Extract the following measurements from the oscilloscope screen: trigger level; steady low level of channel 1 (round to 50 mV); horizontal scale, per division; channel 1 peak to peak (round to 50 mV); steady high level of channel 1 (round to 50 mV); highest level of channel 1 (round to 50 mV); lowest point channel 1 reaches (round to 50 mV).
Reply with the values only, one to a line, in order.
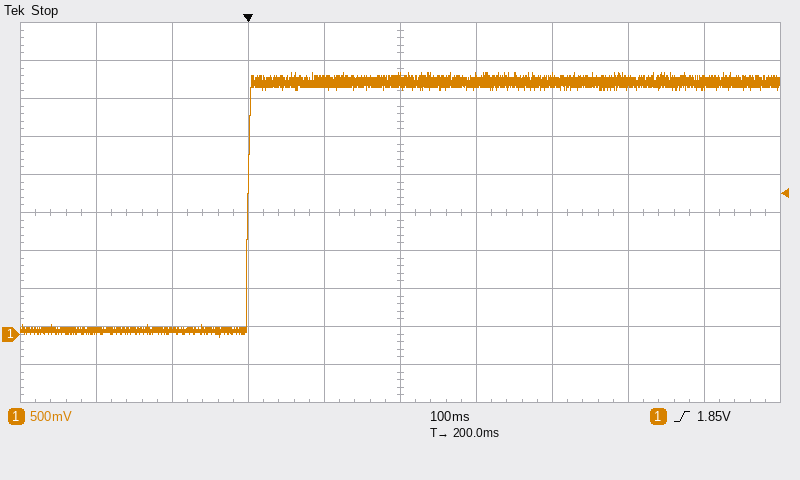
1.85 V
50 mV
100 ms
3.50 V
3.30 V
3.45 V
-50 mV
